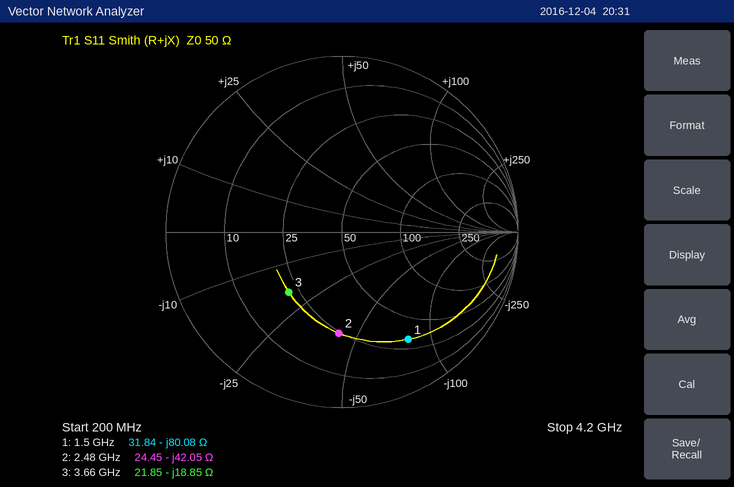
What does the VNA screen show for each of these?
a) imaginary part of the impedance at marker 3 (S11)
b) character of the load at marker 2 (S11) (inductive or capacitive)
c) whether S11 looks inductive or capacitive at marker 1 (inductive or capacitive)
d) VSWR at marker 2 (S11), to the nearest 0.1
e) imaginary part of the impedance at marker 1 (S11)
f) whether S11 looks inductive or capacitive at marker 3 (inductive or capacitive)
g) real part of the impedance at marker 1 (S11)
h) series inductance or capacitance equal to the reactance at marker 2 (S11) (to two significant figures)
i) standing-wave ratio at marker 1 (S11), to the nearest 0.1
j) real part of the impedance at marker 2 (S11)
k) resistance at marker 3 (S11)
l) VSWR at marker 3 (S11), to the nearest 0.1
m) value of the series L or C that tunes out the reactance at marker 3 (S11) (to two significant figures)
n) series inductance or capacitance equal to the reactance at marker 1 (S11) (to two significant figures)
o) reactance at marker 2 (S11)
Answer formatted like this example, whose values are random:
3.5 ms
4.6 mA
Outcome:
-18.85 Ω
capacitive
capacitive
3.7
-80.08 Ω
capacitive
31.84 Ω
1.5 pF
6.1
24.45 Ω
21.85 Ω
2.7
820 pH
1.3 pF
-42.05 Ω
